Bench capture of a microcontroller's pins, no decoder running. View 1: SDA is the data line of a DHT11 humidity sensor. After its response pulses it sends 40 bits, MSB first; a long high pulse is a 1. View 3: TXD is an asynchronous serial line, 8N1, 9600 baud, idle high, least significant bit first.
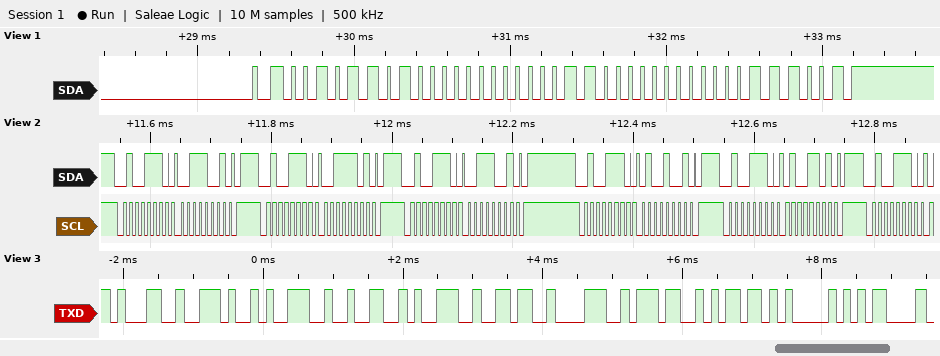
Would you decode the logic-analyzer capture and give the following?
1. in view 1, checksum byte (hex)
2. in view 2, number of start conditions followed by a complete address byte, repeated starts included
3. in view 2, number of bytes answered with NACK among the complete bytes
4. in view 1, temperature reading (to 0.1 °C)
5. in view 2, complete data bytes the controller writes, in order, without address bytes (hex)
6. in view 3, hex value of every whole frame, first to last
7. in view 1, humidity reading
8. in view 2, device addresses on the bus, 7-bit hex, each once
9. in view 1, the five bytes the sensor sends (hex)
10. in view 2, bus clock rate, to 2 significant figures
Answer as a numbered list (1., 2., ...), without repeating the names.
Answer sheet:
1. 0x39
2. 6
3. 0
4. 12.0 °C
5. 39 3D 39 49 4D
6. 0x31 0x2E 0x39 0x32 0x39 0x36 0x38 0x37 0x6D 0x41 0x0D
7. 45 %
8. 0x27
9. 2D 00 0C 00 39
10. 100 kHz
